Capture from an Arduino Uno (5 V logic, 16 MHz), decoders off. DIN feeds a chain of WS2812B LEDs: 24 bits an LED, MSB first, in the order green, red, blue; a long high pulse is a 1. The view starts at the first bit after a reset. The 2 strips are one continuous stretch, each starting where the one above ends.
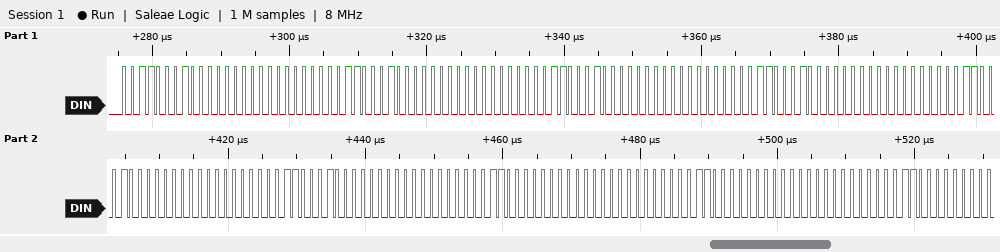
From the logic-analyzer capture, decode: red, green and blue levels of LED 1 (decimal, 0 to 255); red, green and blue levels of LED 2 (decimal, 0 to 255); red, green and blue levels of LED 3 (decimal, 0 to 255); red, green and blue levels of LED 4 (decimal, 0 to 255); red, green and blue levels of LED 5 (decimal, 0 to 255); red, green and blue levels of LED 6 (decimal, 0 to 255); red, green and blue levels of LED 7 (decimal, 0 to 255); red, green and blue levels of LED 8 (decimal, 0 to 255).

0, 49, 0
0, 49, 0
0, 49, 0
0, 49, 0
0, 49, 0
0, 49, 0
0, 48, 0
0, 48, 0
